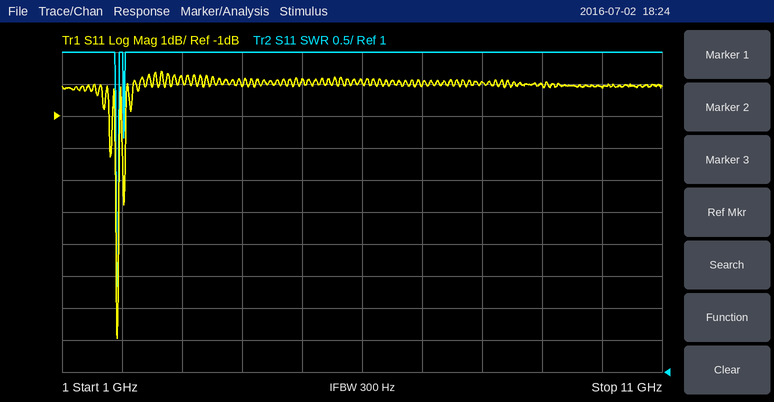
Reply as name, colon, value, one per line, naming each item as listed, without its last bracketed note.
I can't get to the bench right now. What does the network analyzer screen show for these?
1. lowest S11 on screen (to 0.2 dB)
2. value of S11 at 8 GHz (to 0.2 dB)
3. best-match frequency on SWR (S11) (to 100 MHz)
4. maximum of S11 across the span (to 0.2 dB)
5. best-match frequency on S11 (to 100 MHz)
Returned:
lowest S11 on screen: -8.0 dB
value of S11 at 8 GHz: 0.0 dB
best-match frequency on SWR (S11): 1.9 GHz
maximum of S11 across the span: 0.4 dB
best-match frequency on S11: 1.9 GHz
